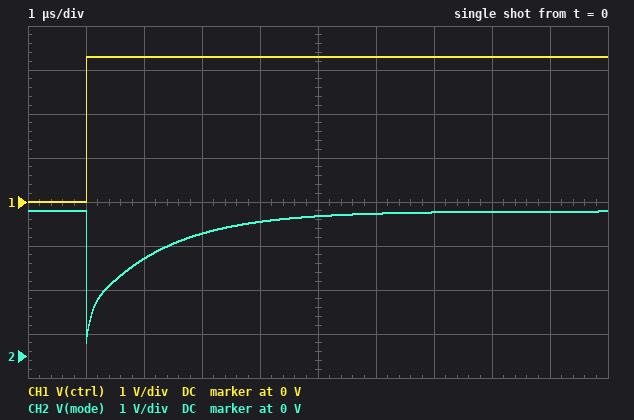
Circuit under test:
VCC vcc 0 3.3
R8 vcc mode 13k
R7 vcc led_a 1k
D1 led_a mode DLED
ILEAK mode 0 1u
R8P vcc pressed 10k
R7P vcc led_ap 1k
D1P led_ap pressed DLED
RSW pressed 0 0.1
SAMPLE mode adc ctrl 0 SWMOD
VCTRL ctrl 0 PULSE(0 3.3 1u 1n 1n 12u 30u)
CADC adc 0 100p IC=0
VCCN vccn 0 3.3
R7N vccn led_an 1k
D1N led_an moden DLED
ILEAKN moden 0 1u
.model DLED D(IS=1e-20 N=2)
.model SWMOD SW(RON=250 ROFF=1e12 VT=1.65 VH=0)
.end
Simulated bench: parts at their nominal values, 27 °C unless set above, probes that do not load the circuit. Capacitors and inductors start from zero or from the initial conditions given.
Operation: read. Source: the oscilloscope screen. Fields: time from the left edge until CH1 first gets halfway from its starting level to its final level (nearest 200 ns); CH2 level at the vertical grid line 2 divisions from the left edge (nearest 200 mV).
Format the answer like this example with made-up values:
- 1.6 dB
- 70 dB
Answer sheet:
- 1.0 µs
- 2.2 V
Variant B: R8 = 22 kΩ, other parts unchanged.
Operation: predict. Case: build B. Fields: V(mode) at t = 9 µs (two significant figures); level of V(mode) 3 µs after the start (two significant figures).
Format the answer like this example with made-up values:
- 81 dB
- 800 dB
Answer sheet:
- 3.2 V
- 2.4 V
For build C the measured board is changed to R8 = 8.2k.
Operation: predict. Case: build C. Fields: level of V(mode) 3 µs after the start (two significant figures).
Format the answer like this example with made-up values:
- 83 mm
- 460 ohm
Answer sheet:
- 3.1 V
